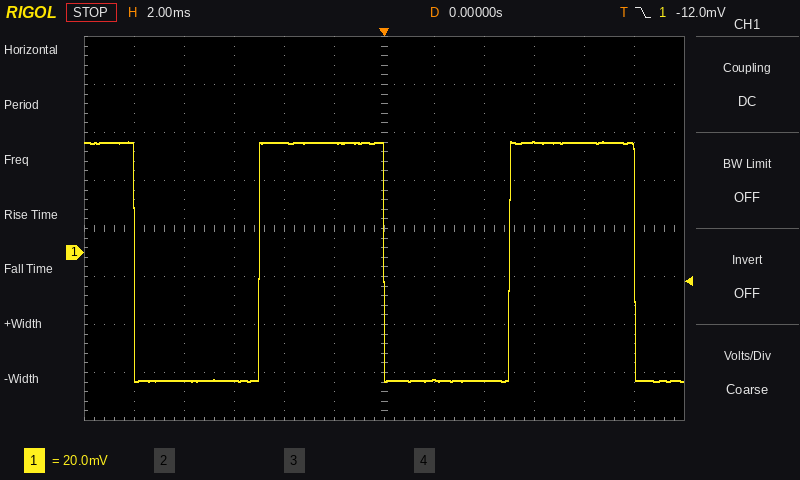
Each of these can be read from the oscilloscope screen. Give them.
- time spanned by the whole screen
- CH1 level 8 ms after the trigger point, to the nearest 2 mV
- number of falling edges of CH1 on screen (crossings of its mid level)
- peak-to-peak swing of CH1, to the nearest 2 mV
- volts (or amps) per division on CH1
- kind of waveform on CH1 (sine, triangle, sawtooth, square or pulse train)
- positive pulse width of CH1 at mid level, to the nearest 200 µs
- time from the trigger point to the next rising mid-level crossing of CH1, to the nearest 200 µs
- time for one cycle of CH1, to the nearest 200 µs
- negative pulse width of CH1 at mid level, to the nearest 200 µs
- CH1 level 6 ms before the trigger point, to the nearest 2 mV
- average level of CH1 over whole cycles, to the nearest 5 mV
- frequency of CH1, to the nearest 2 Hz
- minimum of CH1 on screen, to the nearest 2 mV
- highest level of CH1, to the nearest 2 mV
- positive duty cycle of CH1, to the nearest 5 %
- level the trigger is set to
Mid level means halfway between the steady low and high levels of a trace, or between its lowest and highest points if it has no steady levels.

24 ms
46 mV
3
100 mV
20 mV
square
5.0 ms
5.0 ms
10.0 ms
5.0 ms
-54 mV
-5 mV
100 Hz
-54 mV
46 mV
50 %
-12.0 mV
